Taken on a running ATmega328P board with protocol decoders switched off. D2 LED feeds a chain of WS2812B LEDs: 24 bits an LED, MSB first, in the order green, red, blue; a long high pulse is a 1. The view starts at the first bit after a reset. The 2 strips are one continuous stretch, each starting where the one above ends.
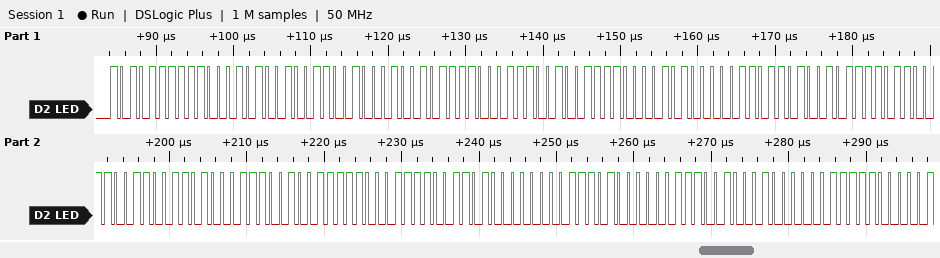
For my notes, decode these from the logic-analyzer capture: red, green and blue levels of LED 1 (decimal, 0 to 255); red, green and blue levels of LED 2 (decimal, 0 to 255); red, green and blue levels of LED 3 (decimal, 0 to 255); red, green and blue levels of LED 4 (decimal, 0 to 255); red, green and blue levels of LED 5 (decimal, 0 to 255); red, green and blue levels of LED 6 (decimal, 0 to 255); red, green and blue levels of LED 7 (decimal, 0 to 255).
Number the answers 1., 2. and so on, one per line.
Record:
1. 197, 175, 38
2. 188, 68, 114
3. 80, 120, 109
4. 102, 47, 102
5. 79, 142, 143
6. 3, 52, 160
7. 32, 114, 124
